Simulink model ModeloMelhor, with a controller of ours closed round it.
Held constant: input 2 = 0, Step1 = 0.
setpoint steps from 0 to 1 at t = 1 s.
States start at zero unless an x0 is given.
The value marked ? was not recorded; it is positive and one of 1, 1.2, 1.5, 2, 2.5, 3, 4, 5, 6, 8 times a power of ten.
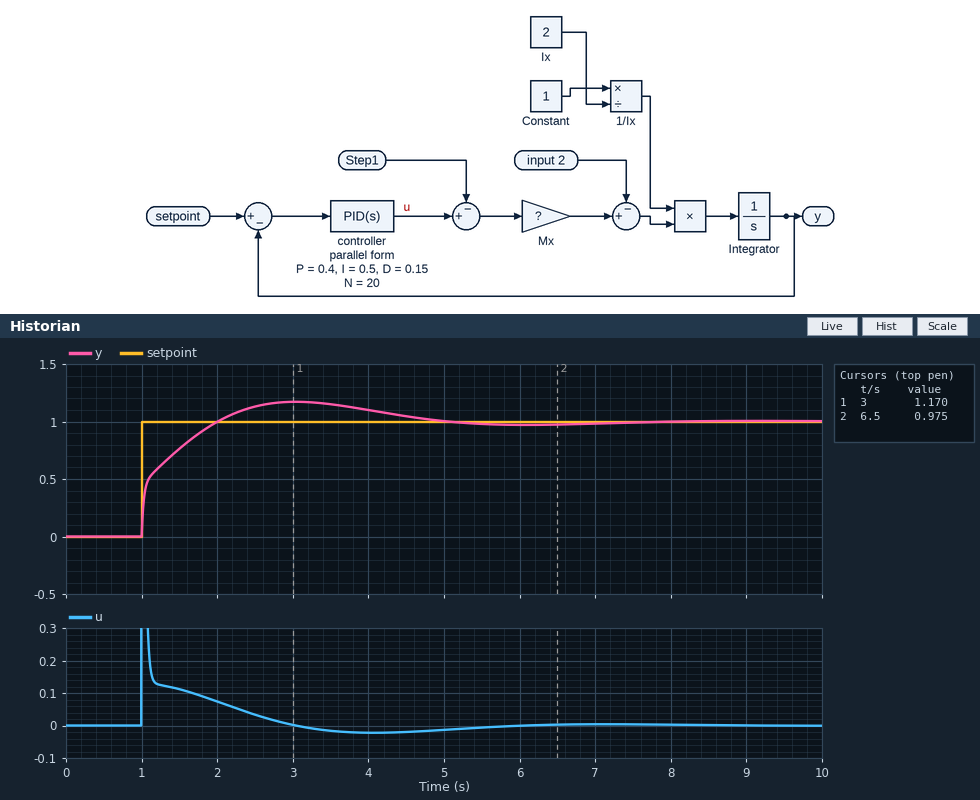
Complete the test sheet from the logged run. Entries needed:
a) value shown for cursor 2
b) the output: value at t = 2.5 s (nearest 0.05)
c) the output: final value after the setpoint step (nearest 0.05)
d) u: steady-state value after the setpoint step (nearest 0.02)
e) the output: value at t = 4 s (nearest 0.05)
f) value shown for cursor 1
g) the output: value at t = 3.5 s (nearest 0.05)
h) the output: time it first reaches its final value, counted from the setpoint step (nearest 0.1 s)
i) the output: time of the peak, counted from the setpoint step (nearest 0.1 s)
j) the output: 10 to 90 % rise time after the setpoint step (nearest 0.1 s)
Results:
0.975
1.15
1.00
0.00
1.10
1.170
1.15
1.0 s
2.0 s
0.8 s
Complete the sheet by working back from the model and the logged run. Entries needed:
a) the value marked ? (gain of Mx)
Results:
10
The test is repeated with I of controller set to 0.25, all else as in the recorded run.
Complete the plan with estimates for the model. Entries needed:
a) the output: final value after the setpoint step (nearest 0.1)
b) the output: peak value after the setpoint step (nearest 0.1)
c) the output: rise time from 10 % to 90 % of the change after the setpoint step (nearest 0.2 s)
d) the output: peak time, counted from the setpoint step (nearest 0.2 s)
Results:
1.0
1.1
1.0 s
2.6 s
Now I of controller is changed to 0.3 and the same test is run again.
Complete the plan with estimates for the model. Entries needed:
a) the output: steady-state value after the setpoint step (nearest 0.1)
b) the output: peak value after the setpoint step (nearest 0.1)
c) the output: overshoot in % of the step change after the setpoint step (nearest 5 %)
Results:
1.0
1.1
15 %
